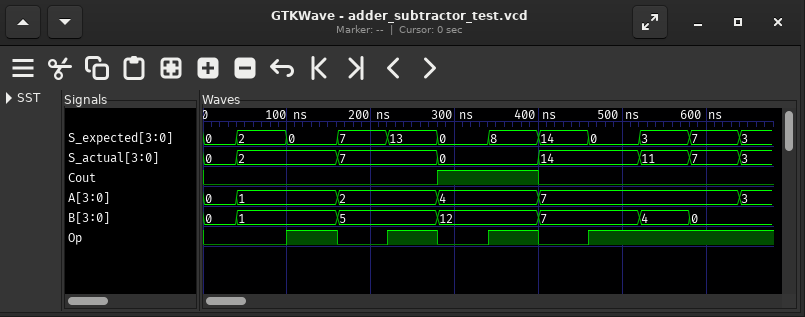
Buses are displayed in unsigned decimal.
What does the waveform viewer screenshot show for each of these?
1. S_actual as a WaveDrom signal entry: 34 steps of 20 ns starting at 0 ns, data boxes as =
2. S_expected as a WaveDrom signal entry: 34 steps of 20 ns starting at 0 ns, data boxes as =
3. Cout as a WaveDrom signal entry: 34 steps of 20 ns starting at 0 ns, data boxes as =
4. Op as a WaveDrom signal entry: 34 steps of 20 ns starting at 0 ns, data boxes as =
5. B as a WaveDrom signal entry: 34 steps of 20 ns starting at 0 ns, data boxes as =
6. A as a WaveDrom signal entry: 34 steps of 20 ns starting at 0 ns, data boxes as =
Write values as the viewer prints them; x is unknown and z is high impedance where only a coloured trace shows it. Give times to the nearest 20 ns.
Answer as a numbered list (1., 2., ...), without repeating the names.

1. {name: 'S_actual', wave: '=.=.....=.....=.....=.....=..=..=.', data: '0 2 7 0 14 11 7 3'}
2. {name: 'S_expected', wave: '=.=..=..=..=..=..=..=..=..=..=..=.', data: '0 2 0 7 13 0 8 14 0 3 7 3'}
3. {name: 'Cout', wave: '0.............1.....0.............'}
4. {name: 'Op', wave: '0....1..0..1..0..1..0..1..........'}
5. {name: 'B', wave: '=.=.....=.....=.....=.....=..=....', data: '0 1 5 12 7 4 0'}
6. {name: 'A', wave: '=.=.....=.....=.....=...........=.', data: '0 1 2 4 7 3'}
